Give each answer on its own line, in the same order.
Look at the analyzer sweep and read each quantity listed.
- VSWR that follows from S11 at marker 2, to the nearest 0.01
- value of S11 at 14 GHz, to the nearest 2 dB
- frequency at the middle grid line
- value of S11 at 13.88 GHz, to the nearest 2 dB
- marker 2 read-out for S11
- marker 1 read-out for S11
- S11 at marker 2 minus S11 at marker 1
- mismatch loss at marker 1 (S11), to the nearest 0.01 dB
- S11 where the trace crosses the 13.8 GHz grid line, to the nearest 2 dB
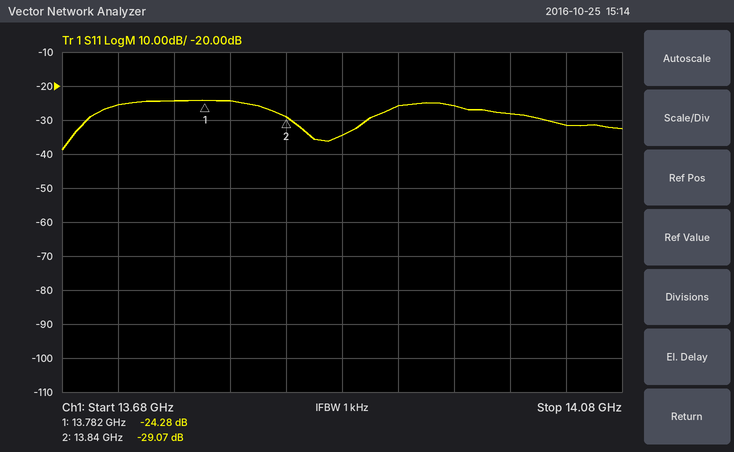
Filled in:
1.07
-28 dB
13.88 GHz
-34 dB
-29.07 dB
-24.28 dB
-4.79 dB
0.02 dB
-24 dB
